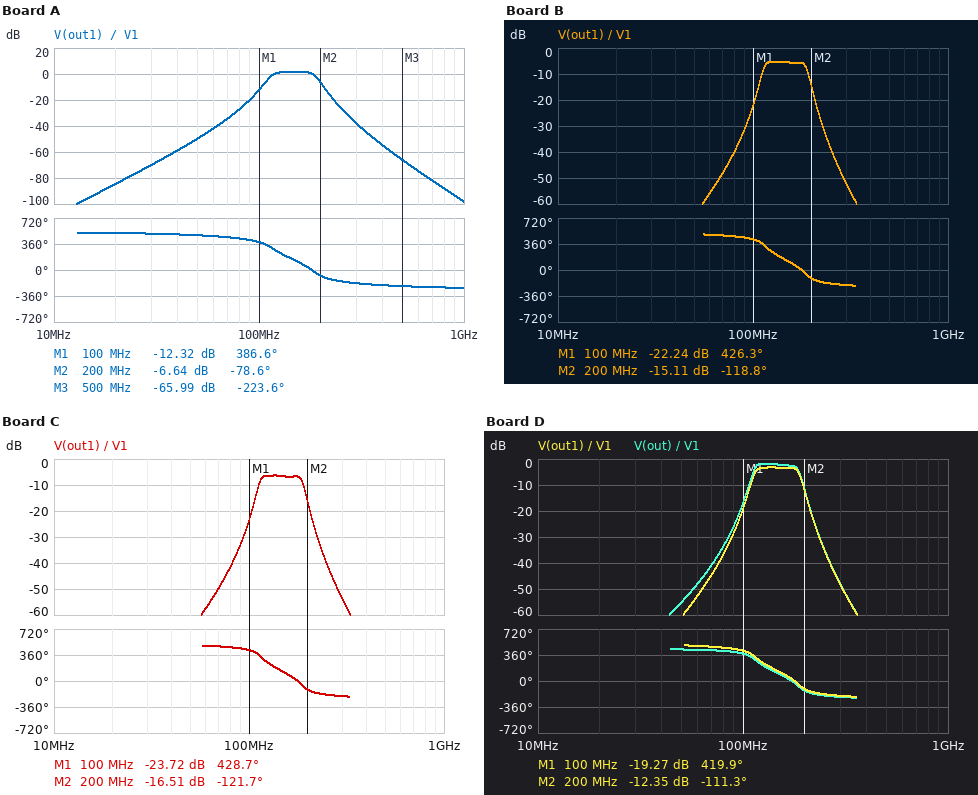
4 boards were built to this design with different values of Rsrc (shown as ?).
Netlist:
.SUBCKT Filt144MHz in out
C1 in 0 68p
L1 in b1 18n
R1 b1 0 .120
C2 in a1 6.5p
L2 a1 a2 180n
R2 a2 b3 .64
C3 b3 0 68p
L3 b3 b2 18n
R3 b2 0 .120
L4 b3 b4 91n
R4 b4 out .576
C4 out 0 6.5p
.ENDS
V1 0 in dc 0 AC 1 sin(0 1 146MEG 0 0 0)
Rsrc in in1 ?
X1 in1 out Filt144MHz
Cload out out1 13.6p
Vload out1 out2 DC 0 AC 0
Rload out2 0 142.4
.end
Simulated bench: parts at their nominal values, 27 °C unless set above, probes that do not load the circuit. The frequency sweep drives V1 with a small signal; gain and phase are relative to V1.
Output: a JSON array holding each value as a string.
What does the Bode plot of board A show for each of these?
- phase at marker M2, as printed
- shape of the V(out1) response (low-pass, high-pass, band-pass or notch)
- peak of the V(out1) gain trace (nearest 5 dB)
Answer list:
["-78.6 deg", "band-pass", "0 dB"]
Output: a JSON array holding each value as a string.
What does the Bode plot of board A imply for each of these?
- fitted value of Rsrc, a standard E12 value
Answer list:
["18 Ω"]
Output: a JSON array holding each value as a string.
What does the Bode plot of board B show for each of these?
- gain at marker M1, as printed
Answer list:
["-22.24 dB"]
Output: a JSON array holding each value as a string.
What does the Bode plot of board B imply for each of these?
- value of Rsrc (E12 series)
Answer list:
["100 Ω"]
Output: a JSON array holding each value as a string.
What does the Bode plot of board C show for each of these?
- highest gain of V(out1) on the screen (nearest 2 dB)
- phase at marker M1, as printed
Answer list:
["-6 dB", "428.7 deg"]
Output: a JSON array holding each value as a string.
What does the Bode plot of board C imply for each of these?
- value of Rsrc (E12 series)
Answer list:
["120 Ω"]
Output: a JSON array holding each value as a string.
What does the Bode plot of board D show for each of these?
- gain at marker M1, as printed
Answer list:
["-19.27 dB"]
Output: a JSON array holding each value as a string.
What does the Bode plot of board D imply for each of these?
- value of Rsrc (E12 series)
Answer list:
["68 Ω"]
